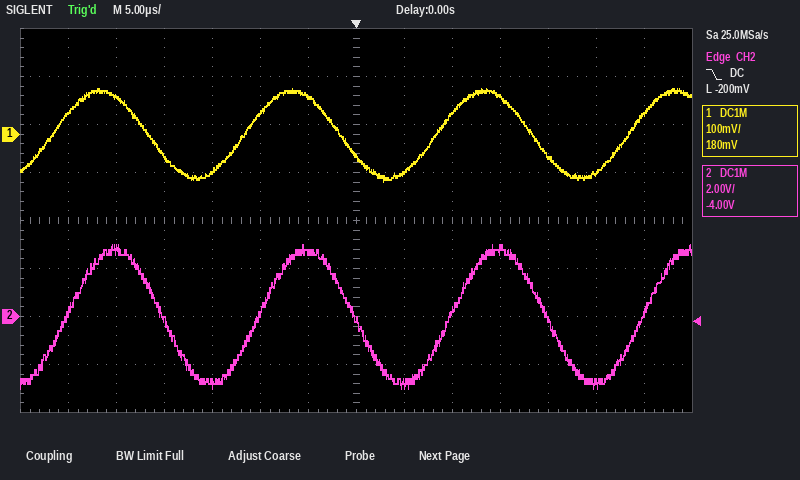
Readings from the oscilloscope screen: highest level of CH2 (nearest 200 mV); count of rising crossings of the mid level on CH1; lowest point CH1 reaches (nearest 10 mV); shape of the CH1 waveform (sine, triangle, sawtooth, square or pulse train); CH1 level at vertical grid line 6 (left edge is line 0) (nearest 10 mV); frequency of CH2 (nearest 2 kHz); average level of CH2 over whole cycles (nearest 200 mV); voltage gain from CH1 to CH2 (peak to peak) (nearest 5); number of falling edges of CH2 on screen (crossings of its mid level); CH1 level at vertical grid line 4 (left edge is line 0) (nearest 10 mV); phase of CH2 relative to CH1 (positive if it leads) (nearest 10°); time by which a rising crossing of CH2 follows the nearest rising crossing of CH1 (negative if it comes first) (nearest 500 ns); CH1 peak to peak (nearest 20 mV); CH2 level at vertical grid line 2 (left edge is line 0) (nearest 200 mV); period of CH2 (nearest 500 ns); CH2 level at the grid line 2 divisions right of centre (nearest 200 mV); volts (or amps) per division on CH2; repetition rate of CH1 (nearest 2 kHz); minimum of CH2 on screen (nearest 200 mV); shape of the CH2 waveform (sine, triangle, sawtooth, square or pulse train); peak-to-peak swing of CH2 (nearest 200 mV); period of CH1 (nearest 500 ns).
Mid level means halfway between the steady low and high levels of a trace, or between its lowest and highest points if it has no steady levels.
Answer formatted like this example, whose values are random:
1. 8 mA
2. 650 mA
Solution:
1. 3.0 V
2. 4
3. -100 mV
4. sine
5. 80 mV
6. 50 kHz
7. 0.0 V
8. 30
9. 3
10. -80 mV
11. -30°
12. +1.5 µs
13. 200 mV
14. 2.8 V
15. 20.0 µs
16. 200 mV
17. 2 V
18. 50 kHz
19. -3.0 V
20. sine
21. 6.0 V
22. 20.0 µs
